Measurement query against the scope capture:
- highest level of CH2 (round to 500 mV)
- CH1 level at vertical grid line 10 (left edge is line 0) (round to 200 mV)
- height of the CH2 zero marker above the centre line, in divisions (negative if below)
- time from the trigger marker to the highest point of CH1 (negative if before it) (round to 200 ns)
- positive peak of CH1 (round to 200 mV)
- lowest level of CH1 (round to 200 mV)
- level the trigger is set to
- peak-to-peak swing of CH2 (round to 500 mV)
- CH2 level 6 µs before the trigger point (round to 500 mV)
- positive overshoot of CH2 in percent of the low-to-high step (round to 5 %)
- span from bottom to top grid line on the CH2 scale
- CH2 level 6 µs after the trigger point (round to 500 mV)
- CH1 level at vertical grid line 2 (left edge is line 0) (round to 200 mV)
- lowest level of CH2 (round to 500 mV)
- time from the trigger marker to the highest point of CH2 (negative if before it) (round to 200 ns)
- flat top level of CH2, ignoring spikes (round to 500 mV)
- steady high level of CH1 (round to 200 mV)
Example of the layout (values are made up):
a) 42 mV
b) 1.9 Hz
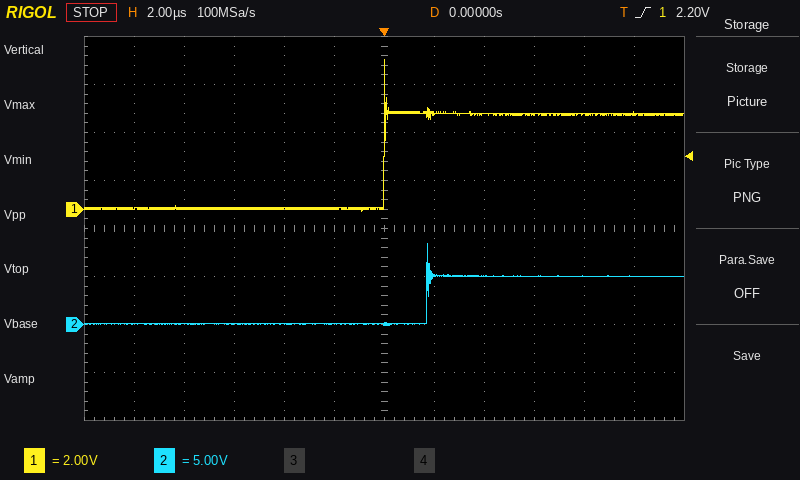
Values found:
a) 8.5 V
b) 4.0 V
c) -2.0 div
d) 0.0 µs
e) 6.2 V
f) 0.0 V
g) 2.20 V
h) 8.5 V
i) 0.0 V
j) 70 %
k) 40 V
l) 5.0 V
m) 0.0 V
n) 0.0 V
o) +1.8 µs
p) 5.0 V
q) 4.0 V
